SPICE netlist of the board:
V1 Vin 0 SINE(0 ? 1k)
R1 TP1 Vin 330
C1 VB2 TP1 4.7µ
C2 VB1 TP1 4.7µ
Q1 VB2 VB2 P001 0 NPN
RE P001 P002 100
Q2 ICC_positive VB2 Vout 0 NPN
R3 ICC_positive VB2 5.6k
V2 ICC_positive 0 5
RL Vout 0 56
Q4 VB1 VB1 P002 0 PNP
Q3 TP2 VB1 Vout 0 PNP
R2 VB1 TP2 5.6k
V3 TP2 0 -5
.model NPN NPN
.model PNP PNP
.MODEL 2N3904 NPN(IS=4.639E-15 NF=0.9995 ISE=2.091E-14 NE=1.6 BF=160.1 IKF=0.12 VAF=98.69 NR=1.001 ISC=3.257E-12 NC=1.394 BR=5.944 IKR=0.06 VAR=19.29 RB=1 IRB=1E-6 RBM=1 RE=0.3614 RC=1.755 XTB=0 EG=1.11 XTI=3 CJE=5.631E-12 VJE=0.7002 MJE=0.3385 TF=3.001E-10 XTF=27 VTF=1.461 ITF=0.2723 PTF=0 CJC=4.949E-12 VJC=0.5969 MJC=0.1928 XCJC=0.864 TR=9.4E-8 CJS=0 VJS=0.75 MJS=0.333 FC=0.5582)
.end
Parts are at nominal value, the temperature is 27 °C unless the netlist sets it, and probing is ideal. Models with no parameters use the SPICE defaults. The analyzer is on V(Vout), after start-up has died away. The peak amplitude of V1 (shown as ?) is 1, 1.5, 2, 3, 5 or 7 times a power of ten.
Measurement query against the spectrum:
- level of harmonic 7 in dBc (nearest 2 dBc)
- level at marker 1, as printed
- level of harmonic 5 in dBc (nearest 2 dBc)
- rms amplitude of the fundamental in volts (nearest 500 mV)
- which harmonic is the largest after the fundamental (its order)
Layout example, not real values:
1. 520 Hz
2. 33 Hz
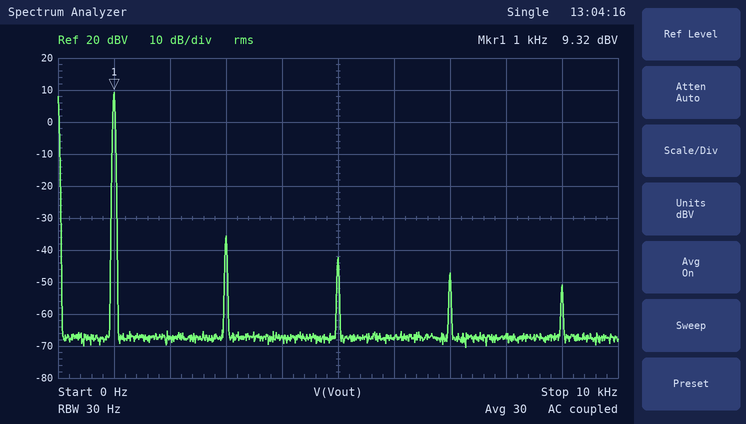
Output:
1. -56 dBc
2. 9.32 dBV
3. -52 dBc
4. 3.0 V
5. 3
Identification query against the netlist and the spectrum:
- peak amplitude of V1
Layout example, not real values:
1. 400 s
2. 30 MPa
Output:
1. 5 V
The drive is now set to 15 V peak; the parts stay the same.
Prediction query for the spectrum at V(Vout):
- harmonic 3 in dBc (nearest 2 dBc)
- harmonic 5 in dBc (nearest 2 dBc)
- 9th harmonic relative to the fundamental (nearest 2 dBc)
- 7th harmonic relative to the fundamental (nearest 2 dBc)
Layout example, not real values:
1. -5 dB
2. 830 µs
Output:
1. -18 dBc
2. -14 dBc
3. -28 dBc
4. -30 dBc
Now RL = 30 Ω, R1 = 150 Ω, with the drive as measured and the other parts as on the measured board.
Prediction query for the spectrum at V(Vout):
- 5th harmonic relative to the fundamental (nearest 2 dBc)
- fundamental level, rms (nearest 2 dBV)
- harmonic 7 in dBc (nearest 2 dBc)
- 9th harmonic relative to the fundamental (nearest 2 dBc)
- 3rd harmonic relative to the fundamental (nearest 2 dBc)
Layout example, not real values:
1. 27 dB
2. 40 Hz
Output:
1. -46 dBc
2. 10 dBV
3. -50 dBc
4. -54 dBc
5. -40 dBc
